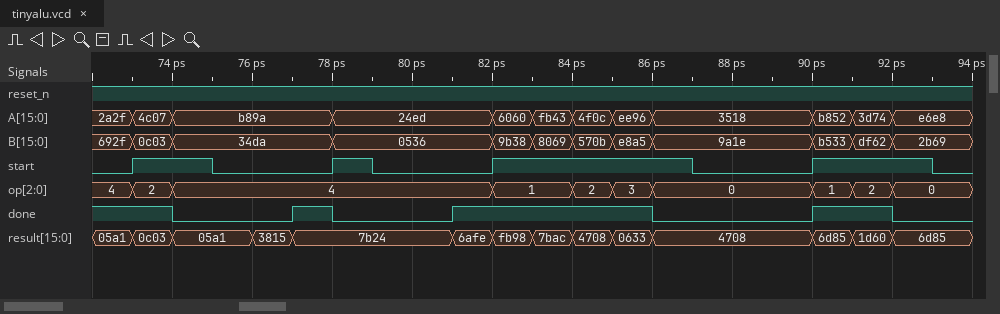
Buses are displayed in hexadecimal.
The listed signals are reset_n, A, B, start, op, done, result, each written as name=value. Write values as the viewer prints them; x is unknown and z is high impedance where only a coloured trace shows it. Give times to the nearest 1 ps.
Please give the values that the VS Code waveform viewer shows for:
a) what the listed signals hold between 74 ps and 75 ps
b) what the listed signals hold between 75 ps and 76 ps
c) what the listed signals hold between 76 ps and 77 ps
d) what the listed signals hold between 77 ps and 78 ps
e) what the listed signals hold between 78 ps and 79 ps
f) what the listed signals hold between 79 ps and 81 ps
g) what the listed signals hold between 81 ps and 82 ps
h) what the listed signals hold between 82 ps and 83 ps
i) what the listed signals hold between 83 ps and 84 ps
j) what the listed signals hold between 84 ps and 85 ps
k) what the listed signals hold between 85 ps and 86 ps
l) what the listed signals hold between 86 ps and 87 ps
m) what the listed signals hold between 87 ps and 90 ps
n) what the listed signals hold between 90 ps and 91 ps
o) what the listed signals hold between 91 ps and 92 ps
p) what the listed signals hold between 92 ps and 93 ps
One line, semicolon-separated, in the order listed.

reset_n=1, A=b89a, B=34da, start=1, op=4, done=0, result=05a1; reset_n=1, A=b89a, B=34da, start=0, op=4, done=0, result=05a1; reset_n=1, A=b89a, B=34da, start=0, op=4, done=0, result=3815; reset_n=1, A=b89a, B=34da, start=0, op=4, done=1, result=7b24; reset_n=1, A=24ed, B=0536, start=1, op=4, done=0, result=7b24; reset_n=1, A=24ed, B=0536, start=0, op=4, done=0, result=7b24; reset_n=1, A=24ed, B=0536, start=0, op=4, done=1, result=6afe; reset_n=1, A=6060, B=9b38, start=1, op=1, done=1, result=fb98; reset_n=1, A=fb43, B=8069, start=1, op=1, done=1, result=7bac; reset_n=1, A=4f0c, B=570b, start=1, op=2, done=1, result=4708; reset_n=1, A=ee96, B=e8a5, start=1, op=3, done=1, result=0633; reset_n=1, A=3518, B=9a1e, start=1, op=0, done=0, result=4708; reset_n=1, A=3518, B=9a1e, start=0, op=0, done=0, result=4708; reset_n=1, A=b852, B=b533, start=1, op=1, done=1, result=6d85; reset_n=1, A=3d74, B=df62, start=1, op=2, done=1, result=1d60; reset_n=1, A=e6e8, B=2b69, start=1, op=0, done=0, result=6d85
